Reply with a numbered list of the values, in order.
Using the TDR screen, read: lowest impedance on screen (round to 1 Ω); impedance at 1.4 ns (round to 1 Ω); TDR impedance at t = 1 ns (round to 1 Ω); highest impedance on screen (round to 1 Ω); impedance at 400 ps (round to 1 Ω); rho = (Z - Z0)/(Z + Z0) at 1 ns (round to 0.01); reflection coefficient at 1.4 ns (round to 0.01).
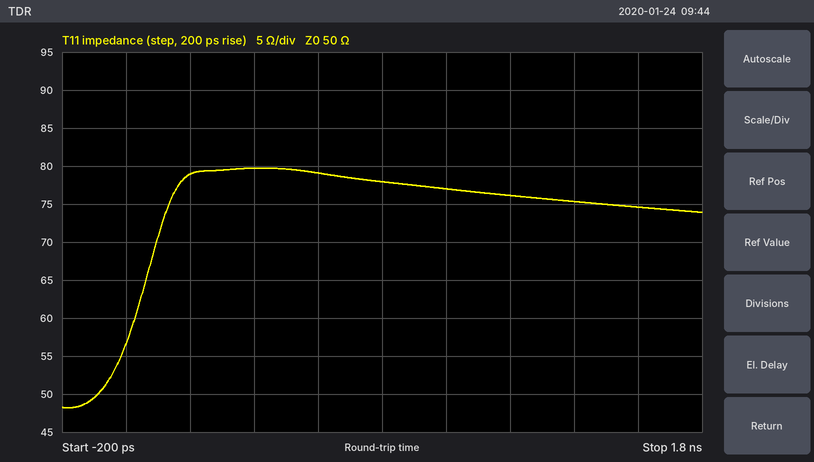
1. 48 Ω
2. 75 Ω
3. 77 Ω
4. 80 Ω
5. 80 Ω
6. +0.21
7. +0.20
